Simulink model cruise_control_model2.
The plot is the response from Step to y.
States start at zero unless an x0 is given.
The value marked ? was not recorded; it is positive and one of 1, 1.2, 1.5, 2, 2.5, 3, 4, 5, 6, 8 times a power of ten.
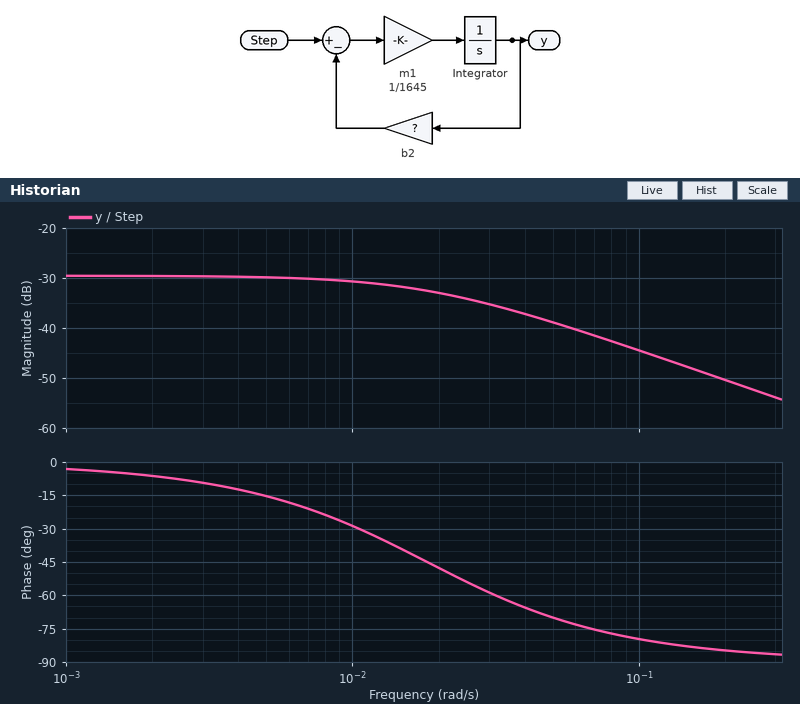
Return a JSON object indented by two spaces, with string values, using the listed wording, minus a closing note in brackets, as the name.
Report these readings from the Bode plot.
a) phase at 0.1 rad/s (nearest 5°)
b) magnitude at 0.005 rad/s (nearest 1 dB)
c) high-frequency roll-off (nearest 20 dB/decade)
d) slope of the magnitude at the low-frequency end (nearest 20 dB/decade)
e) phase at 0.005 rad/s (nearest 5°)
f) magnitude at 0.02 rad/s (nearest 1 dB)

{
  "phase at 0.1 rad/s": "-80°",
  "magnitude at 0.005 rad/s": "-30 dB",
  "high-frequency roll-off": "-20 dB/decade",
  "slope of the magnitude at the low-frequency end": "0 dB/decade",
  "phase at 0.005 rad/s": "-15°",
  "magnitude at 0.02 rad/s": "-33 dB"
}
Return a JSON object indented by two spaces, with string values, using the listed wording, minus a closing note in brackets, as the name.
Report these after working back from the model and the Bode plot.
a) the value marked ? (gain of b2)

{
  "the value marked ?": "30"
}
